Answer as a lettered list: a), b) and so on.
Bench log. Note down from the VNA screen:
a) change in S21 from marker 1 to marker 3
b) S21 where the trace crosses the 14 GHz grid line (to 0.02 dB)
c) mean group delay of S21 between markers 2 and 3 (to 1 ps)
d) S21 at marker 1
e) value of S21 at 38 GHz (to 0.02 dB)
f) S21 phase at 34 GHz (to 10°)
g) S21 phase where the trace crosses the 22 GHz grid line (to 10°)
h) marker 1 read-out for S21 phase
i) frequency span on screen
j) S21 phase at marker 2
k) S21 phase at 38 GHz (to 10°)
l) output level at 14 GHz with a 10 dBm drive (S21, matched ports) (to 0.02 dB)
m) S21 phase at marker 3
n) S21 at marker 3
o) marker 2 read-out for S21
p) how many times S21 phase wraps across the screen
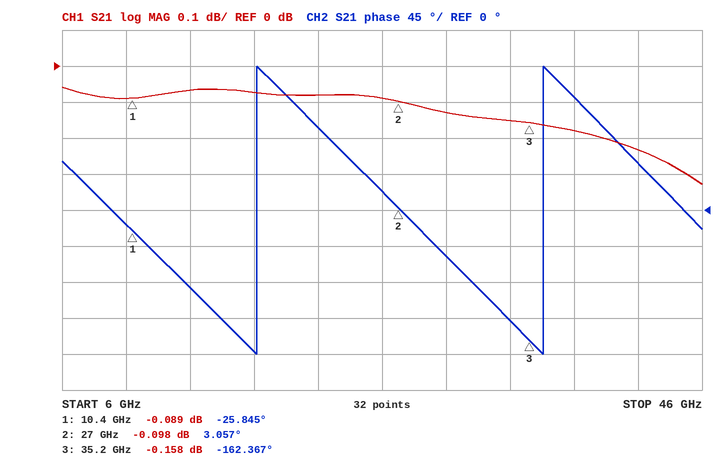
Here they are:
a) -0.069 dB
b) -0.06 dB
c) 56 ps
d) -0.089 dB
e) -0.18 dB
f) -140°
g) 100°
h) -25.845°
i) 40 GHz
j) 3.057°
k) 140°
l) 9.94 dBm
m) -162.367°
n) -0.158 dB
o) -0.098 dB
p) 2
